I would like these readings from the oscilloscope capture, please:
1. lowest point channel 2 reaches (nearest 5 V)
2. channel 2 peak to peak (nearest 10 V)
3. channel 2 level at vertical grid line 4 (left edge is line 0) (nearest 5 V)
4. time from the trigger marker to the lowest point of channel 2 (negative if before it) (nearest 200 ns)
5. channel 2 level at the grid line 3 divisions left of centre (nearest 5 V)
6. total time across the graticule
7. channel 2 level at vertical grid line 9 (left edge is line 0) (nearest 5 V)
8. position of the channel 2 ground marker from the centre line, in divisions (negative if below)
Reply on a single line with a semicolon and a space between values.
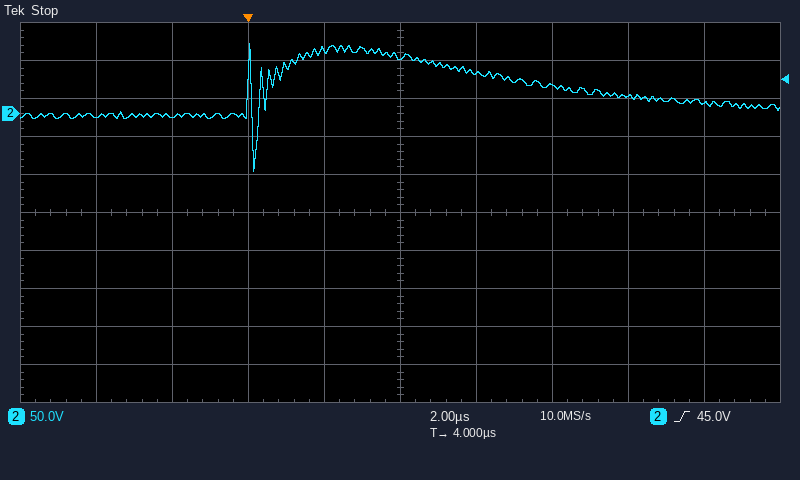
-75 V; 170 V; 85 V; +200 ns; -5 V; 20 µs; 15 V; +2.6 div
